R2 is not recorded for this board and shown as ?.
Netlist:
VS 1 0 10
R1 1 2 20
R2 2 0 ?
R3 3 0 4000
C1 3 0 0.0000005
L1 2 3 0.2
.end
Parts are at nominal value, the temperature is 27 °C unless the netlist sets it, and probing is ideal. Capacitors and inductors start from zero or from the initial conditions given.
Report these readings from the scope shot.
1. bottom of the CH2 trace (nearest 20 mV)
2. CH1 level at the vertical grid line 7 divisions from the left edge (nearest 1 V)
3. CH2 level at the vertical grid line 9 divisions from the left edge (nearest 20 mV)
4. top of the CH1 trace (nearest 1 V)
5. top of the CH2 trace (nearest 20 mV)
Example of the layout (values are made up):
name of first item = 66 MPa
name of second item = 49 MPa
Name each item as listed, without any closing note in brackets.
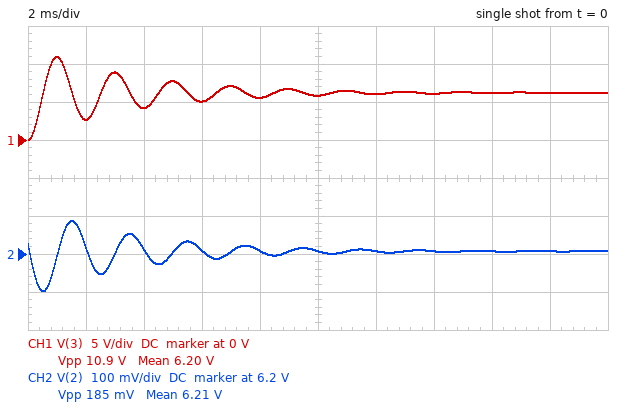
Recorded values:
bottom of the CH2 trace = 6.10 V
CH1 level at the vertical grid line 7 divisions from the left edge = 6 V
CH2 level at the vertical grid line 9 divisions from the left edge = 6.20 V
top of the CH1 trace = 11 V
top of the CH2 trace = 6.28 V
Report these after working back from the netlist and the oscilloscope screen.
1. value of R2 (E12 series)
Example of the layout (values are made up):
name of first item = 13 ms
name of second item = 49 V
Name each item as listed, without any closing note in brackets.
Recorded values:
value of R2 = 33 Ω
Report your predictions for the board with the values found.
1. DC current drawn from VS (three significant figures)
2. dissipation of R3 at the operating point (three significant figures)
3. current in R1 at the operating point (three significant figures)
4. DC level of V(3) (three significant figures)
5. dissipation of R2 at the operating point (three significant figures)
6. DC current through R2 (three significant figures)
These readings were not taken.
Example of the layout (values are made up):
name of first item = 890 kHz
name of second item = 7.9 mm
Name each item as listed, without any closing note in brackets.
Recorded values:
DC current drawn from VS = 190 mA
dissipation of R3 at the operating point = 9.63 mW
current in R1 at the operating point = 190 mA
DC level of V(3) = 6.21 V
dissipation of R2 at the operating point = 1.17 W
DC current through R2 = 188 mA
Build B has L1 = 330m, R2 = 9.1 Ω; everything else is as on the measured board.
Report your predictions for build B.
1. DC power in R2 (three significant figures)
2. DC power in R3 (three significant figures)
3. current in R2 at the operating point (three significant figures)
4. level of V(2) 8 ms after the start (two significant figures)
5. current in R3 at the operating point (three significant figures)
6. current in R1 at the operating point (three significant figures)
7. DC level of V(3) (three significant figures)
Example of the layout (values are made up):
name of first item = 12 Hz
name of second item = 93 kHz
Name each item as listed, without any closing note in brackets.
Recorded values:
DC power in R2 = 1.07 W
DC power in R3 = 2.44 mW
current in R2 at the operating point = 343 mA
level of V(2) 8 ms after the start = 3.1 V
current in R3 at the operating point = 781 µA
current in R1 at the operating point = 344 mA
DC level of V(3) = 3.12 V
